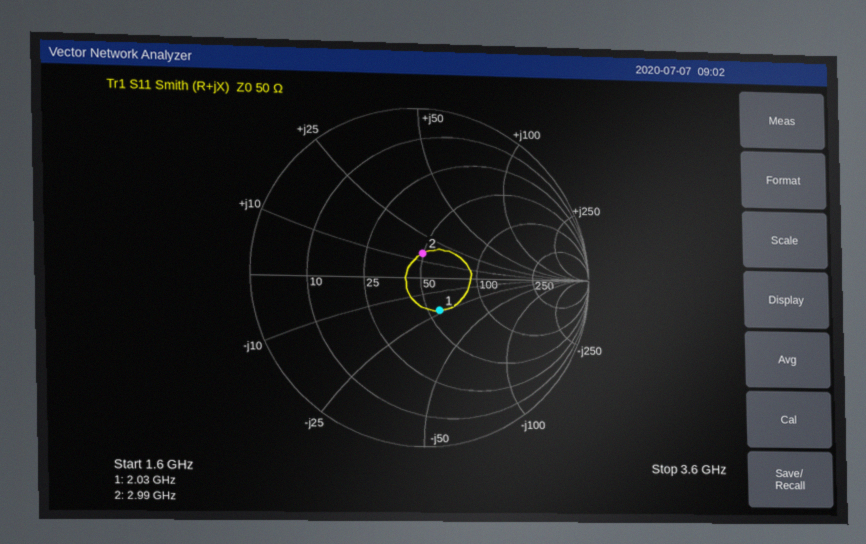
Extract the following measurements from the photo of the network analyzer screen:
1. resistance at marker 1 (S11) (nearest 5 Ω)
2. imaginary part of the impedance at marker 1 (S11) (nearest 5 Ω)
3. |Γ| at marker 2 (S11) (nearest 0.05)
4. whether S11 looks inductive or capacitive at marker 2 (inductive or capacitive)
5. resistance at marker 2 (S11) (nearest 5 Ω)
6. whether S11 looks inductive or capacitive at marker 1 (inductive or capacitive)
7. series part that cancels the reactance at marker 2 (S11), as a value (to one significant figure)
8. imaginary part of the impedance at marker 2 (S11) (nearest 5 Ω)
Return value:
55 Ω
-25 Ω
0.15
inductive
50 Ω
capacitive
4 pF
+15 Ω
